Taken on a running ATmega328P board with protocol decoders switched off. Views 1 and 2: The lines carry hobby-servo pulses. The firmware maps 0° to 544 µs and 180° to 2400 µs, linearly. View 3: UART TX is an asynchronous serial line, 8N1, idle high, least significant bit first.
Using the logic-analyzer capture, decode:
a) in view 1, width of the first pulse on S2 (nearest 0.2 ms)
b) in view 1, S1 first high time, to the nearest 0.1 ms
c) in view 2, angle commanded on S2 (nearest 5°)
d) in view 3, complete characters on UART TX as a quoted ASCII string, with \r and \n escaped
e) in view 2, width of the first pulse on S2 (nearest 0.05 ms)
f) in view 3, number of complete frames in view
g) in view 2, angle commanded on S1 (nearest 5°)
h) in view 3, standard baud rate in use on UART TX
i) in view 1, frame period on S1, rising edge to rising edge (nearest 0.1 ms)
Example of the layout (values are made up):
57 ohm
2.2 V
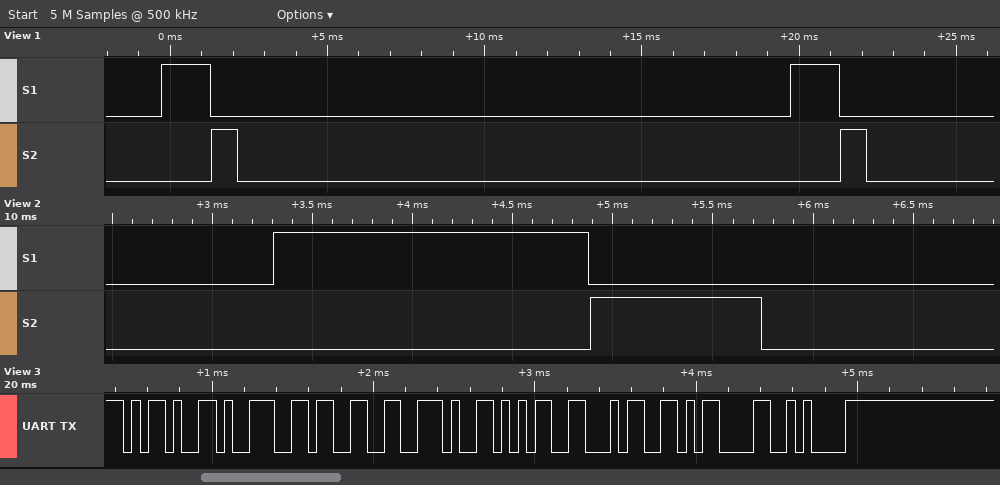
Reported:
0.8 ms
1.6 ms
30°
"-93.54\r\n"
0.85 ms
8
100°
19200 baud
20.0 ms
